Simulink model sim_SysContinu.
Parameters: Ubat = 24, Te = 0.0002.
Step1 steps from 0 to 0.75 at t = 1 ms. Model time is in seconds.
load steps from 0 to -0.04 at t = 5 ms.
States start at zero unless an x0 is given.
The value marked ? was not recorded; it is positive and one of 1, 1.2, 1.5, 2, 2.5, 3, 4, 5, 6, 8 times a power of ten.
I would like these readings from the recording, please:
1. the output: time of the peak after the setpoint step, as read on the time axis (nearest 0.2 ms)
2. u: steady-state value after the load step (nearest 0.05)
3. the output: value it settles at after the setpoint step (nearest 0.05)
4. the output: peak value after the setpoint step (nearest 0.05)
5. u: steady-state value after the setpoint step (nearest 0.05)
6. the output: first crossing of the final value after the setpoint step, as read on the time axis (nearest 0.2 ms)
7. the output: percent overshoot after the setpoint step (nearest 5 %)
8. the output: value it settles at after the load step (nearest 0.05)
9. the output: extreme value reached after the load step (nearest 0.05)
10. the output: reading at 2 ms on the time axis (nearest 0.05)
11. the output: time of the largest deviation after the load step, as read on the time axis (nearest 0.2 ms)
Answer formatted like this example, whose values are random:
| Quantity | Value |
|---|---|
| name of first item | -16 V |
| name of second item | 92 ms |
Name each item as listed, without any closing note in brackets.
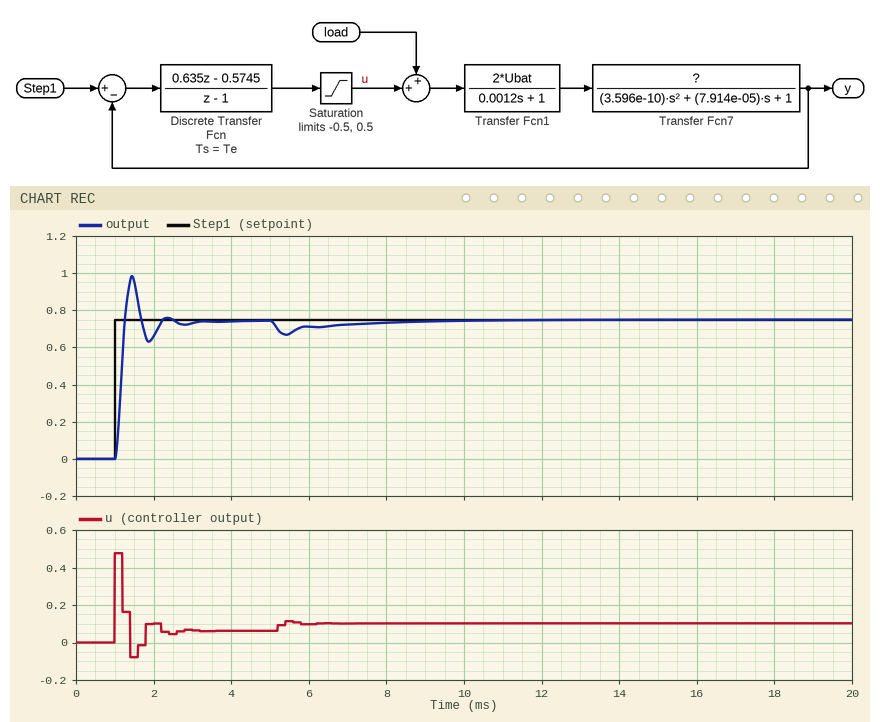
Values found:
| Quantity | Value |
|---|---|
| the output: time of the peak after the setpoint step, as read on the time axis | 1.4 ms |
| u: steady-state value after the load step | 0.10 |
| the output: value it settles at after the setpoint step | 0.75 |
| the output: peak value after the setpoint step | 1.00 |
| u: steady-state value after the setpoint step | 0.05 |
| the output: first crossing of the final value after the setpoint step, as read on the time axis | 1.2 ms |
| the output: percent overshoot after the setpoint step | 30 % |
| the output: value it settles at after the load step | 0.75 |
| the output: extreme value reached after the load step | 0.65 |
| the output: reading at 2 ms on the time axis | 0.65 |
| the output: time of the largest deviation after the load step, as read on the time axis | 5.4 ms |
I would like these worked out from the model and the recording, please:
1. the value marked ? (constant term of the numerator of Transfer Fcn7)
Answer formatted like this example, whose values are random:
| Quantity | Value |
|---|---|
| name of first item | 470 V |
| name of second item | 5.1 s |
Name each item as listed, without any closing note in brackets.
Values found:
| Quantity | Value |
|---|---|
| the value marked ? | 0.25 |
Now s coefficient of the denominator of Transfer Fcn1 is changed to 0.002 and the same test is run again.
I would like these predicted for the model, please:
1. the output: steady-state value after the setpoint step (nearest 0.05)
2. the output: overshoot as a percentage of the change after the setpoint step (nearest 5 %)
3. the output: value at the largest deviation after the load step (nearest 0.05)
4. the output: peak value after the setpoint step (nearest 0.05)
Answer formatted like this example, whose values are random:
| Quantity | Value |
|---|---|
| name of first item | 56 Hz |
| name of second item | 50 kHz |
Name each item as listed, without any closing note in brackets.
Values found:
| Quantity | Value |
|---|---|
| the output: steady-state value after the setpoint step | 0.75 |
| the output: overshoot as a percentage of the change after the setpoint step | 15 % |
| the output: value at the largest deviation after the load step | 0.70 |
| the output: peak value after the setpoint step | 0.85 |
